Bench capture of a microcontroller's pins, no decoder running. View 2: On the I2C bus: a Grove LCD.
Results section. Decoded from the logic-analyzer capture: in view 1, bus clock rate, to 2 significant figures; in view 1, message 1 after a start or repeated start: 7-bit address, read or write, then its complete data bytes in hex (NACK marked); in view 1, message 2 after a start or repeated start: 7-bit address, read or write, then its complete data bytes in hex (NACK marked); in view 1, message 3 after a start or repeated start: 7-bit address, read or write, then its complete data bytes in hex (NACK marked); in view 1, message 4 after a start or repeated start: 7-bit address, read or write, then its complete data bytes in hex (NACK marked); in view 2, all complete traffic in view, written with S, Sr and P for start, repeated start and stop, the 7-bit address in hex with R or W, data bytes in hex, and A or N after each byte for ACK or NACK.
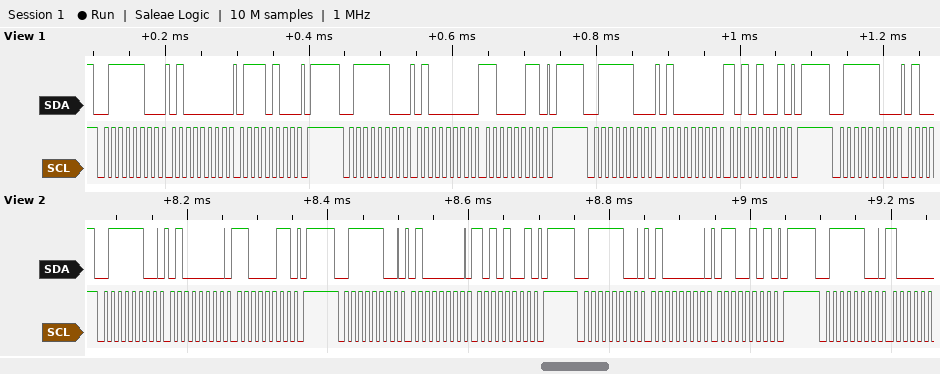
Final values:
100 kHz
0x3E write: 40 74
0x3E write: 40 C3
0x3E write: 40 A9
0x3E write
S 3EW A 40 A C3 A P S 3EW A 40 A A9 A P S 3EW A 40 A 65 A P S 3EW A
